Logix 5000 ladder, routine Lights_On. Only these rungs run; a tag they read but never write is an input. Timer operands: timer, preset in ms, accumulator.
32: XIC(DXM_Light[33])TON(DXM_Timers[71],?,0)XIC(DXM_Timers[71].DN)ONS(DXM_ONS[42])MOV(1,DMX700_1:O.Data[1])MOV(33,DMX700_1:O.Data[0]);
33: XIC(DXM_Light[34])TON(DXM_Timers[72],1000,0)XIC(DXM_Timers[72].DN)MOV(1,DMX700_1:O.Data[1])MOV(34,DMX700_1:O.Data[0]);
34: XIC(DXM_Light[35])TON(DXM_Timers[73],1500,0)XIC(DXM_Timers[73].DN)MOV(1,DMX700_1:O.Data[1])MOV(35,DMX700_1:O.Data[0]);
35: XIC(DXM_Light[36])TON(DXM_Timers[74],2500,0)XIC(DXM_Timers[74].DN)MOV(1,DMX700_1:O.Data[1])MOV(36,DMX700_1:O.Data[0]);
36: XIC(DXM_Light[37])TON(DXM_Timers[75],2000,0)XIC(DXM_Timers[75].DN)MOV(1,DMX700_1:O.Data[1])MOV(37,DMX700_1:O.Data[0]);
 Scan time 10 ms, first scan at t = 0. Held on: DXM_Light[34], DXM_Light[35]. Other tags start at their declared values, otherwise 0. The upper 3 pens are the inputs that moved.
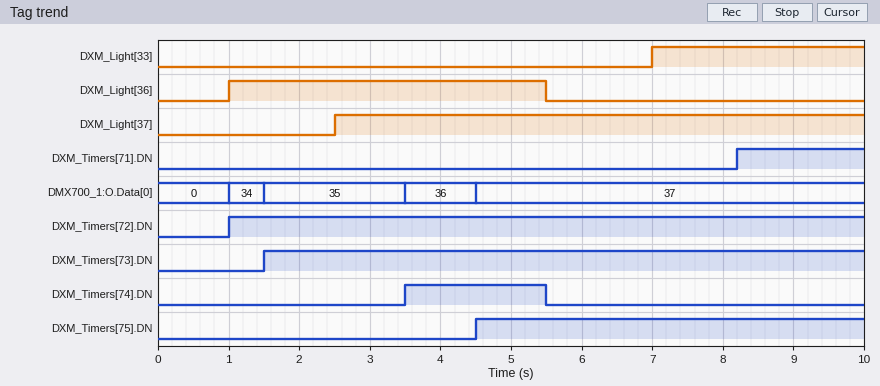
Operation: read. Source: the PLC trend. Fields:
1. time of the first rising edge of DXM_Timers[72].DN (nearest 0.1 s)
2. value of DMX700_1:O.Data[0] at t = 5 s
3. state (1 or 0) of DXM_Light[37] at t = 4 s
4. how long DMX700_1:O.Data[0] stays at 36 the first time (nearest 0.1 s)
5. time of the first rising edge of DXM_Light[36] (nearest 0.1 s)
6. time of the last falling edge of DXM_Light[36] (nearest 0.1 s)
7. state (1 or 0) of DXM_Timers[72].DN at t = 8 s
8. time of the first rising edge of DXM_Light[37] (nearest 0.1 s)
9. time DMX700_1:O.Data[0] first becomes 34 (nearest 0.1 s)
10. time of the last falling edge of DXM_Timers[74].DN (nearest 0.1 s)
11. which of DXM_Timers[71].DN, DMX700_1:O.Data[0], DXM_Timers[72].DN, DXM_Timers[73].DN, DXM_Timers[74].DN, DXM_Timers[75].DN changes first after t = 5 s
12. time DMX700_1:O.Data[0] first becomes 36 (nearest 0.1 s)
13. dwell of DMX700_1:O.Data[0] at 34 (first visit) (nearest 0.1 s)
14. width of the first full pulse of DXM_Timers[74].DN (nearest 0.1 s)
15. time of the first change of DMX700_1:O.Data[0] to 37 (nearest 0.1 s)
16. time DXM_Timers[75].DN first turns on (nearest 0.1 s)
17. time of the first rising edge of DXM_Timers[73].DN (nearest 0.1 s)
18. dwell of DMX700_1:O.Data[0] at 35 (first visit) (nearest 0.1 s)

1.0 s
37
1
1.0 s
1.0 s
5.5 s
1
2.5 s
1.0 s
5.5 s
DXM_Timers[74].DN
3.5 s
0.5 s
2.0 s
4.5 s
4.5 s
1.5 s
2.0 s
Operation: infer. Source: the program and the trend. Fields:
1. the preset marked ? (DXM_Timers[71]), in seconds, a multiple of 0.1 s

1.2 s
